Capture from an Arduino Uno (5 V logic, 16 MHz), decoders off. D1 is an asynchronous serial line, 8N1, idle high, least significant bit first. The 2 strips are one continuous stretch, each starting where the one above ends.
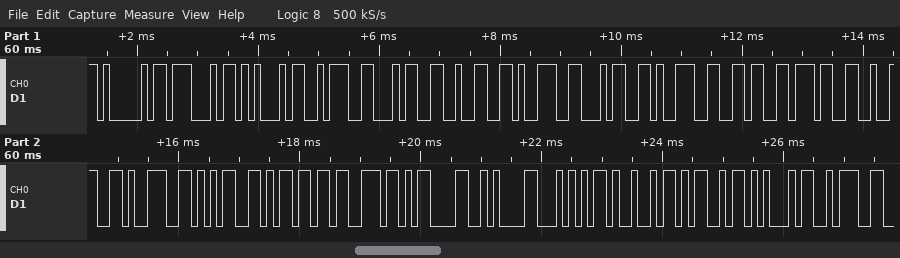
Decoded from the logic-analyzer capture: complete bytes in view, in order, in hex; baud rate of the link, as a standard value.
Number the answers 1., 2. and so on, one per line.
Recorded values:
1. 41 47 45 3A 34 32 39 34 39 36 37 32 39 35 6D 73 0D 0A 54 49 4D 45 3A
2. 9600 baud
